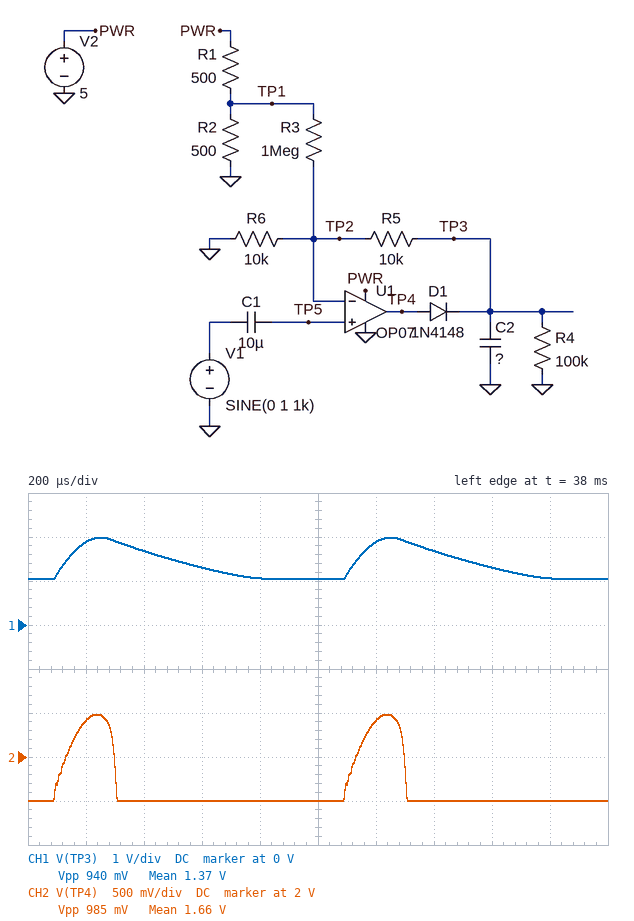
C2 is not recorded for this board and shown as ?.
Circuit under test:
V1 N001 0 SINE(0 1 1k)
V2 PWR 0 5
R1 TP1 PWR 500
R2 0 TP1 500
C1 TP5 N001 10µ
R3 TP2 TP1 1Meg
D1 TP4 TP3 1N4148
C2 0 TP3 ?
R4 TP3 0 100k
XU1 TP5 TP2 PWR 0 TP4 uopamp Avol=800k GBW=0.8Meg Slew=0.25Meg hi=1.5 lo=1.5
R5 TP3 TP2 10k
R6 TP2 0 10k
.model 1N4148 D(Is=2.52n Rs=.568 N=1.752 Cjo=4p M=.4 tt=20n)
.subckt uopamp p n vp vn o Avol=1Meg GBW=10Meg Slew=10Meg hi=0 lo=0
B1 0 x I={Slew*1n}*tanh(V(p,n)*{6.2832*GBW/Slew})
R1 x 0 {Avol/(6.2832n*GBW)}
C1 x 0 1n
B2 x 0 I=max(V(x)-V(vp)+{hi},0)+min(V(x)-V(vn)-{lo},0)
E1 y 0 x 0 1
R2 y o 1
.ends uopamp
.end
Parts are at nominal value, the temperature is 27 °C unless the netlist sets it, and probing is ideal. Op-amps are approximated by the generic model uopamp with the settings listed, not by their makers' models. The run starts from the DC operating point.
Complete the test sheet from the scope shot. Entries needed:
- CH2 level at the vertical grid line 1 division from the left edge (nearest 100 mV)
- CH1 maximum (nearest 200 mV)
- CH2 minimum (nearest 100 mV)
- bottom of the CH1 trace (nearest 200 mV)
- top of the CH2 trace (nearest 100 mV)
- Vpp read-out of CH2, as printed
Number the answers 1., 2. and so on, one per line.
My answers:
1. 2.4 V
2. 2.0 V
3. 1.5 V
4. 1.0 V
5. 2.5 V
6. 985 mV
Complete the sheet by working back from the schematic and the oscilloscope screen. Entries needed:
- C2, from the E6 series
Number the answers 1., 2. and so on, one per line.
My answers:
1. 47 nF
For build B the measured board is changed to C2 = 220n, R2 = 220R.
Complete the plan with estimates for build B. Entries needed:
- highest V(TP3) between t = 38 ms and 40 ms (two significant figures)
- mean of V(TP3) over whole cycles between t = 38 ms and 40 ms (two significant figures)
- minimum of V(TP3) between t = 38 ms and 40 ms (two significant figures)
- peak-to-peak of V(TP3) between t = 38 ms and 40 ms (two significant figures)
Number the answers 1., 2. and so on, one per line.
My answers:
1. 2.0 V
2. 1.8 V
3. 1.6 V
4. 430 mV
